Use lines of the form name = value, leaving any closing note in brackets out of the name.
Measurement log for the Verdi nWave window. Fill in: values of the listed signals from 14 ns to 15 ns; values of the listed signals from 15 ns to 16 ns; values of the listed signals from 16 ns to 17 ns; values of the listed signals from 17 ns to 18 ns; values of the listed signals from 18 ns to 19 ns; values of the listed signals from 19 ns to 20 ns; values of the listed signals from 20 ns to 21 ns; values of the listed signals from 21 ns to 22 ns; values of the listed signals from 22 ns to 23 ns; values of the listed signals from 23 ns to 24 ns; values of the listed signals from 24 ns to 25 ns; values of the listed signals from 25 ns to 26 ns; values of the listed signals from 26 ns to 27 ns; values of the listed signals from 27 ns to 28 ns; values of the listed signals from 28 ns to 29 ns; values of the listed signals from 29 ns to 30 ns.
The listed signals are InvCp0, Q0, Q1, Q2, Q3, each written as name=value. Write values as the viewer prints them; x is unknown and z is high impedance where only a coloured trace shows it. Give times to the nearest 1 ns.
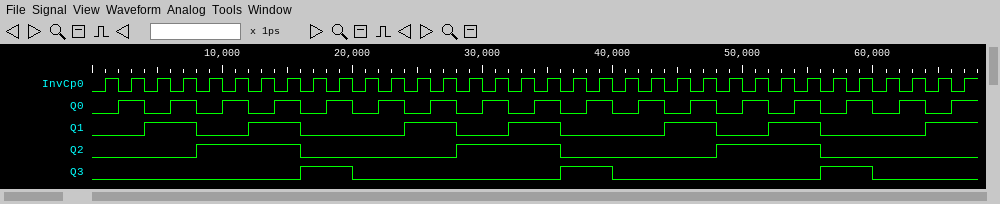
values of the listed signals from 14 ns to 15 ns = InvCp0=0, Q0=1, Q1=1, Q2=1, Q3=0
values of the listed signals from 15 ns to 16 ns = InvCp0=1, Q0=1, Q1=1, Q2=1, Q3=0
values of the listed signals from 16 ns to 17 ns = InvCp0=0, Q0=0, Q1=0, Q2=0, Q3=1
values of the listed signals from 17 ns to 18 ns = InvCp0=1, Q0=0, Q1=0, Q2=0, Q3=1
values of the listed signals from 18 ns to 19 ns = InvCp0=0, Q0=1, Q1=0, Q2=0, Q3=1
values of the listed signals from 19 ns to 20 ns = InvCp0=1, Q0=1, Q1=0, Q2=0, Q3=1
values of the listed signals from 20 ns to 21 ns = InvCp0=0, Q0=0, Q1=0, Q2=0, Q3=0
values of the listed signals from 21 ns to 22 ns = InvCp0=1, Q0=0, Q1=0, Q2=0, Q3=0
values of the listed signals from 22 ns to 23 ns = InvCp0=0, Q0=1, Q1=0, Q2=0, Q3=0
values of the listed signals from 23 ns to 24 ns = InvCp0=1, Q0=1, Q1=0, Q2=0, Q3=0
values of the listed signals from 24 ns to 25 ns = InvCp0=0, Q0=0, Q1=1, Q2=0, Q3=0
values of the listed signals from 25 ns to 26 ns = InvCp0=1, Q0=0, Q1=1, Q2=0, Q3=0
values of the listed signals from 26 ns to 27 ns = InvCp0=0, Q0=1, Q1=1, Q2=0, Q3=0
values of the listed signals from 27 ns to 28 ns = InvCp0=1, Q0=1, Q1=1, Q2=0, Q3=0
values of the listed signals from 28 ns to 29 ns = InvCp0=0, Q0=0, Q1=0, Q2=1, Q3=0
values of the listed signals from 29 ns to 30 ns = InvCp0=1, Q0=0, Q1=0, Q2=1, Q3=0
